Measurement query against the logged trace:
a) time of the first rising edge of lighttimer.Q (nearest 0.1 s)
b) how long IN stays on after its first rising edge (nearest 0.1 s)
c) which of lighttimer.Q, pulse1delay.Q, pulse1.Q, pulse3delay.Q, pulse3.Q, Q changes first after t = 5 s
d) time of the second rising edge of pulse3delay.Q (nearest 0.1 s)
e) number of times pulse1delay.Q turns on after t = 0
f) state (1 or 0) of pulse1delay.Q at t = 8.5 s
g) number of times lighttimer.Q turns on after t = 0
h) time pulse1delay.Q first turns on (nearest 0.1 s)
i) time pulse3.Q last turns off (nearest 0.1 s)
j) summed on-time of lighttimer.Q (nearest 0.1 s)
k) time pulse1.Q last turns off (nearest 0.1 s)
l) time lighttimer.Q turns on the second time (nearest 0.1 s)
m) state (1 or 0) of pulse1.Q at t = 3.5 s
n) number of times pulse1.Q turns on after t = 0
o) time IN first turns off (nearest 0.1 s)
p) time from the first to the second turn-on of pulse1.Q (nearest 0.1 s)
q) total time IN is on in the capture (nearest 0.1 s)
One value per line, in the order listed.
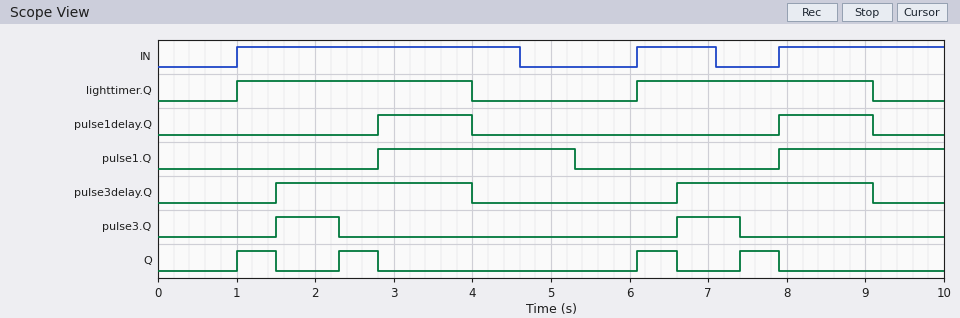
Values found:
1.0 s
3.6 s
pulse1.Q
6.6 s
2
1
2
2.8 s
7.4 s
6.0 s
5.3 s
6.1 s
1
2
4.6 s
5.1 s
6.7 s
